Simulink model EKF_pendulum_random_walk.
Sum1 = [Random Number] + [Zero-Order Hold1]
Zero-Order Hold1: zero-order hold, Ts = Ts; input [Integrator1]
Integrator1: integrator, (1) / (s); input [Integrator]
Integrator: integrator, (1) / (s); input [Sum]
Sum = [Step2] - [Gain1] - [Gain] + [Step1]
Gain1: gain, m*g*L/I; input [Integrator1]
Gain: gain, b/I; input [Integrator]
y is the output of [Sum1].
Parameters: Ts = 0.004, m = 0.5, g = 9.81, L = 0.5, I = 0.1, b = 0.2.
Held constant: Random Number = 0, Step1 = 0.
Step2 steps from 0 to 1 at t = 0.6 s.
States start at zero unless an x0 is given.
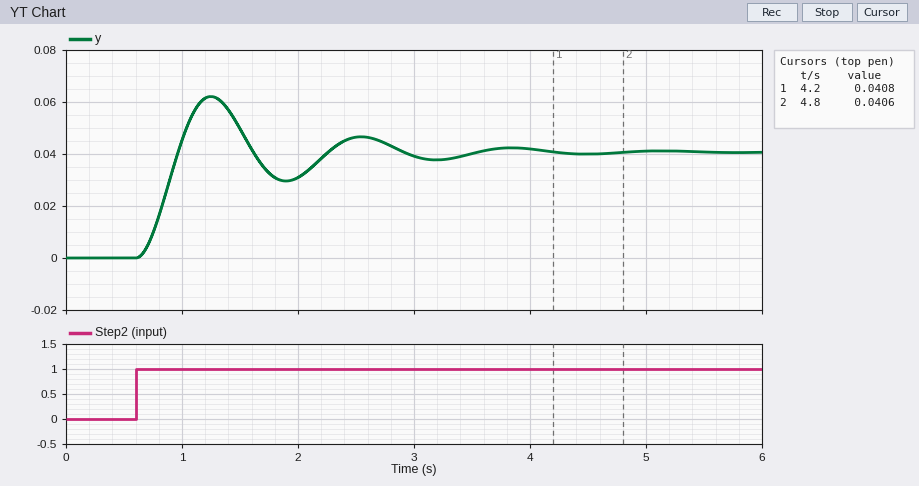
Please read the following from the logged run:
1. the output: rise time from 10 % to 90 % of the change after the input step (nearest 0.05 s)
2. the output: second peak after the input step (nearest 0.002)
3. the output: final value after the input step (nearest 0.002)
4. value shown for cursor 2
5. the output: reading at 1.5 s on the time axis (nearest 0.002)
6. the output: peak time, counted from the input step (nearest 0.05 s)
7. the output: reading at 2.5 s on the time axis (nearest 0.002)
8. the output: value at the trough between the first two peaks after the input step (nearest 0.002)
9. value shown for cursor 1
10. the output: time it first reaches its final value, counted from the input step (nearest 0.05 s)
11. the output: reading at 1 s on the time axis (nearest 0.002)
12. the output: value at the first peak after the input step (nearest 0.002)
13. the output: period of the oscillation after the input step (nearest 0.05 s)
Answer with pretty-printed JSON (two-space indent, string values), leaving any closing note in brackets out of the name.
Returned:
{
  "the output: rise time from 10 % to 90 % of the change after the input step": "0.25 s",
  "the output: second peak after the input step": "0.046",
  "the output: final value after the input step": "0.040",
  "value shown for cursor 2": "0.0406",
  "the output: reading at 1.5 s on the time axis": "0.050",
  "the output: peak time, counted from the input step": "0.65 s",
  "the output: reading at 2.5 s on the time axis": "0.046",
  "the output: value at the trough between the first two peaks after the input step": "0.030",
  "value shown for cursor 1": "0.0408",
  "the output: time it first reaches its final value, counted from the input step": "0.35 s",
  "the output: reading at 1 s on the time axis": "0.046",
  "the output: value at the first peak after the input step": "0.062",
  "the output: period of the oscillation after the input step": "1.30 s"
}
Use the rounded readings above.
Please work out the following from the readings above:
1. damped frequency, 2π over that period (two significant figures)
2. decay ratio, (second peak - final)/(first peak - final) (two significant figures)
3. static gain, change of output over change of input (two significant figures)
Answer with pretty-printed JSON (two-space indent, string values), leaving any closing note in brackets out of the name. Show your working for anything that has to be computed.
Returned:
{
  "damped frequency, 2π over that period": "2π / 1.3 = 4.8 rad/s",
  "decay ratio, (second peak - final)/(first peak - final)": "(0.046 - 0.04) / (0.062 - 0.04) = 0.27",
  "static gain, change of output over change of input": "(0.04 - 0) / (1 - 0) = 0.040"
}
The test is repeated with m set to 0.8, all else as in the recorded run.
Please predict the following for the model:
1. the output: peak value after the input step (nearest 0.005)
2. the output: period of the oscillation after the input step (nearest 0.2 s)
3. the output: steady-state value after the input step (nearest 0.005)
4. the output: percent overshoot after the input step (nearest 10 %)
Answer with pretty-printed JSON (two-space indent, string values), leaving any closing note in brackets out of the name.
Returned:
{
  "the output: peak value after the input step": "0.040",
  "the output: period of the oscillation after the input step": "1.0 s",
  "the output: steady-state value after the input step": "0.025",
  "the output: percent overshoot after the input step": "60 %"
}
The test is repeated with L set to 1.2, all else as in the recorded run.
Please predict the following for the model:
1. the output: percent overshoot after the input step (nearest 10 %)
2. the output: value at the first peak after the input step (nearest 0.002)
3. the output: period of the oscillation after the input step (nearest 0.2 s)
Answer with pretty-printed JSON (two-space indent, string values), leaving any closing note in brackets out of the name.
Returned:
{
  "the output: percent overshoot after the input step": "70 %",
  "the output: value at the first peak after the input step": "0.028",
  "the output: period of the oscillation after the input step": "0.8 s"
}
